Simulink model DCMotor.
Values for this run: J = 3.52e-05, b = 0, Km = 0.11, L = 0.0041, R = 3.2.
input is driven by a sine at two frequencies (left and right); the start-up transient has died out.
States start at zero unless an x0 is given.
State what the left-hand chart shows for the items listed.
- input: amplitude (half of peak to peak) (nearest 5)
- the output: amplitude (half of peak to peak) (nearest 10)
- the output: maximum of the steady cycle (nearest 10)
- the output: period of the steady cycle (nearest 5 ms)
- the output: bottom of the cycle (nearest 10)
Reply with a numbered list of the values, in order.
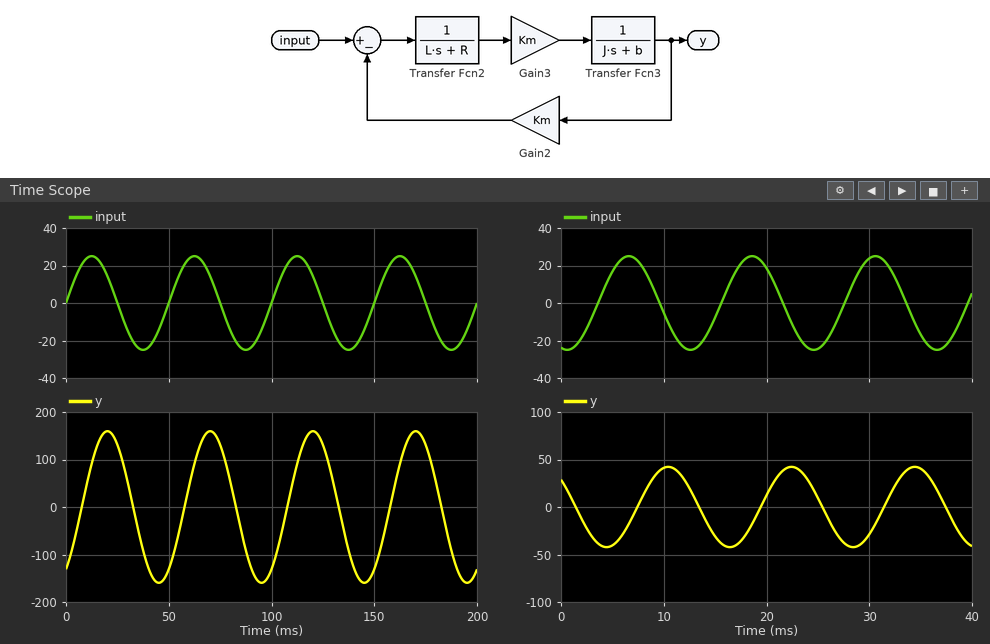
1. 25
2. 160
3. 160
4. 50 ms
5. -160
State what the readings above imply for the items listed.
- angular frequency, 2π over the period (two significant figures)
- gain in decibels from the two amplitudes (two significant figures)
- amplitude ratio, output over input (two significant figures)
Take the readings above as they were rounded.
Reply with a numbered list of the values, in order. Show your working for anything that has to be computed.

1. 2π / 50 = 0.13 rad/ms
2. 20 log10(160 / 25) = 16 dB
3. 160 / 25 = 6.4
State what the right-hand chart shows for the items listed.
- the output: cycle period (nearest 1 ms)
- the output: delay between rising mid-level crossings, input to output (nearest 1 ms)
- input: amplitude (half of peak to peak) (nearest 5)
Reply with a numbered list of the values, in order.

1. 12 ms
2. 4 ms
3. 25
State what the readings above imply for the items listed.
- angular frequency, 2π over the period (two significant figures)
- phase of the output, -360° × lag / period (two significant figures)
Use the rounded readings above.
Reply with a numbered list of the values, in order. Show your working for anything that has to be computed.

1. 2π / 12 = 0.52 rad/ms
2. -360 × 4 / 12 = -120°
